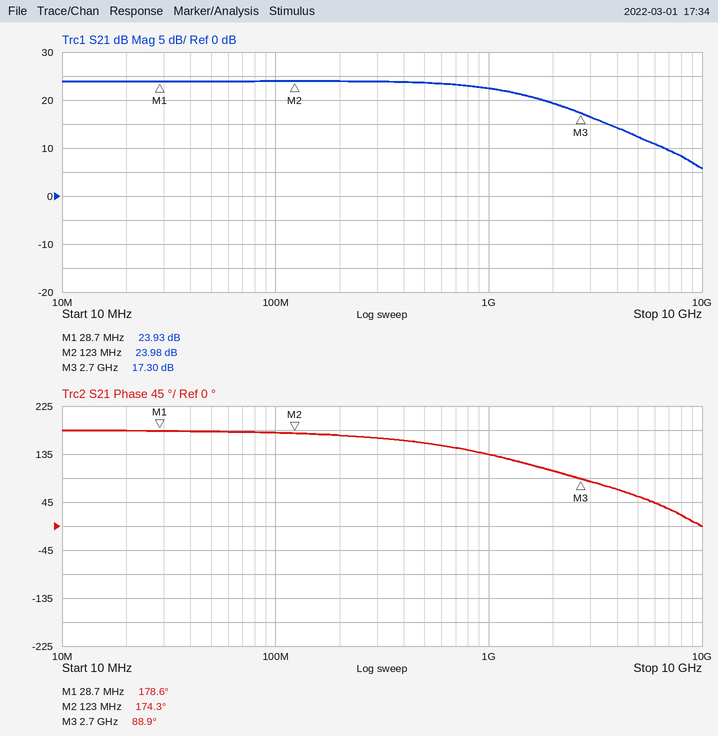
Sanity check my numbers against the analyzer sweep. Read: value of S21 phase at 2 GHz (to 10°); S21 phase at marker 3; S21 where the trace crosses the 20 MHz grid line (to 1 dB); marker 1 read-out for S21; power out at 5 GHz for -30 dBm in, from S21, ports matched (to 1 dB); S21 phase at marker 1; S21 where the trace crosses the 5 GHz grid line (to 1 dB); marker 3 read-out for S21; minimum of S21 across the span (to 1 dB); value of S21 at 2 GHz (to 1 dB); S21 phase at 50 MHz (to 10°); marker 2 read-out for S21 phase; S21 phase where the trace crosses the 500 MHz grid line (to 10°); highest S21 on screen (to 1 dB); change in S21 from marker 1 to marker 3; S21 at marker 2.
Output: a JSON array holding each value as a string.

["100°", "88.9°", "24 dB", "23.93 dB", "-18 dBm", "178.6°", "12 dB", "17.30 dB", "6 dB", "19 dB", "180°", "174.3°", "160°", "24 dB", "-6.63 dB", "23.98 dB"]
